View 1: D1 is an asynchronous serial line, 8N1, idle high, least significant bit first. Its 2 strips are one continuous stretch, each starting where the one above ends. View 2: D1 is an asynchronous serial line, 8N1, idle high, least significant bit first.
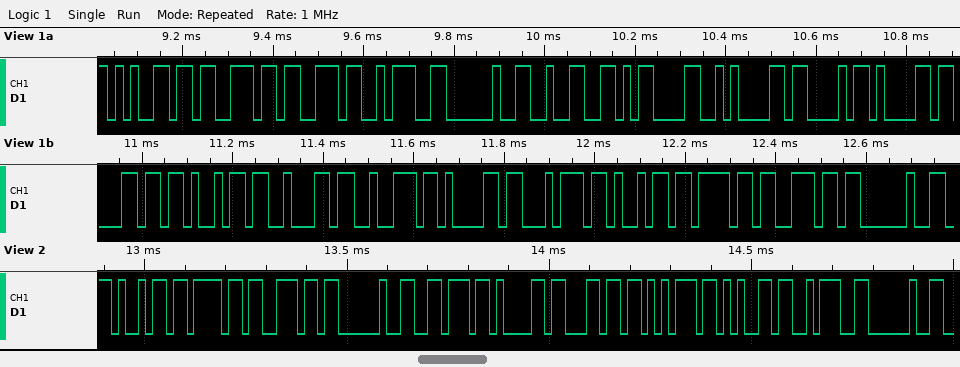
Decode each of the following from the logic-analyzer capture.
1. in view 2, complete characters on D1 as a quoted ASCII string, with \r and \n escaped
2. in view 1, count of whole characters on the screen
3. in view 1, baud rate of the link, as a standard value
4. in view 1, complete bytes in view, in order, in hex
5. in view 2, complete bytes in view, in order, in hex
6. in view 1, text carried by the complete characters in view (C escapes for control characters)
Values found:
"ion value: "
20
57600 baud
65 73 73 3A 20 32 0D 0A 43 61 6C 69 62 72 61 74 69 6F 6E 20
69 6F 6E 20 76 61 6C 75 65 3A 20
"ess: 2\r\nCalibration "
